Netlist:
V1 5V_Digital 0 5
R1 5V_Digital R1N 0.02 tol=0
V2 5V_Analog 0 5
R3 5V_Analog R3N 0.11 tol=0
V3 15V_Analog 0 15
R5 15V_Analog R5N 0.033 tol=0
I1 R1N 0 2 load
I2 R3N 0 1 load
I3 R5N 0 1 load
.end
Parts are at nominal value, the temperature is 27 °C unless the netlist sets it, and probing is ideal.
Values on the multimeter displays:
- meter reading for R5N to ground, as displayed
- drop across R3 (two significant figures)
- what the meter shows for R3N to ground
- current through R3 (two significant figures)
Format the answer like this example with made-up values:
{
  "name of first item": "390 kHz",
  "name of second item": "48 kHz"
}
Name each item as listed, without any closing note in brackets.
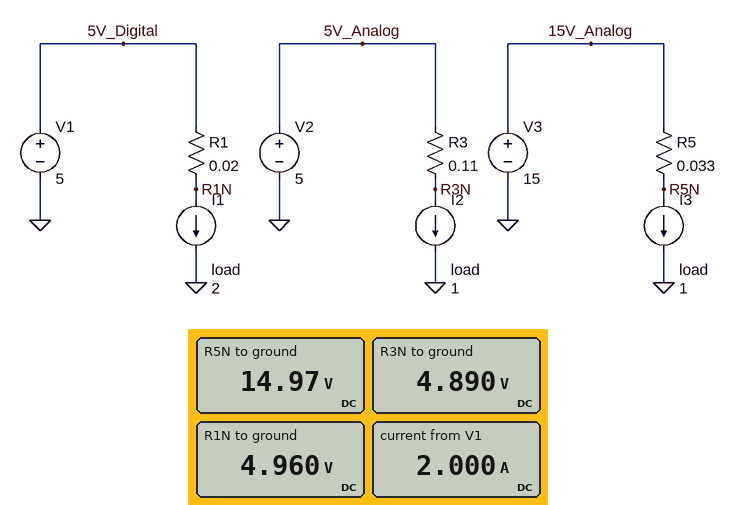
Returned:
{
  "meter reading for R5N to ground, as displayed": "14.97 V",
  "drop across R3": "110 mV",
  "what the meter shows for R3N to ground": "4.890 V",
  "current through R3": "1.0 A"
}
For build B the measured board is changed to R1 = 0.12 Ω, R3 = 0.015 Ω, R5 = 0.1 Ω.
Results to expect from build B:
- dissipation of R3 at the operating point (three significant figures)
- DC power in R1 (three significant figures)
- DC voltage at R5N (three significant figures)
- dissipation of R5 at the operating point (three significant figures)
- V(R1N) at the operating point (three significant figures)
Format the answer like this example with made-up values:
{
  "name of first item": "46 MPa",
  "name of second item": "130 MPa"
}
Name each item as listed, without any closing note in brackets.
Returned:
{
  "dissipation of R3 at the operating point": "15.0 mW",
  "DC power in R1": "480 mW",
  "DC voltage at R5N": "14.9 V",
  "dissipation of R5 at the operating point": "100 mW",
  "V(R1N) at the operating point": "4.76 V"
}
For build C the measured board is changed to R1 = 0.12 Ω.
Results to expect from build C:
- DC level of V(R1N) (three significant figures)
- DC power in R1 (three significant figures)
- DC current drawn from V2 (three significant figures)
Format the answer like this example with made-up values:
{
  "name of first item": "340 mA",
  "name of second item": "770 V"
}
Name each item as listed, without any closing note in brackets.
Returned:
{
  "DC level of V(R1N)": "4.76 V",
  "DC power in R1": "480 mW",
  "DC current drawn from V2": "1.00 A"
}
